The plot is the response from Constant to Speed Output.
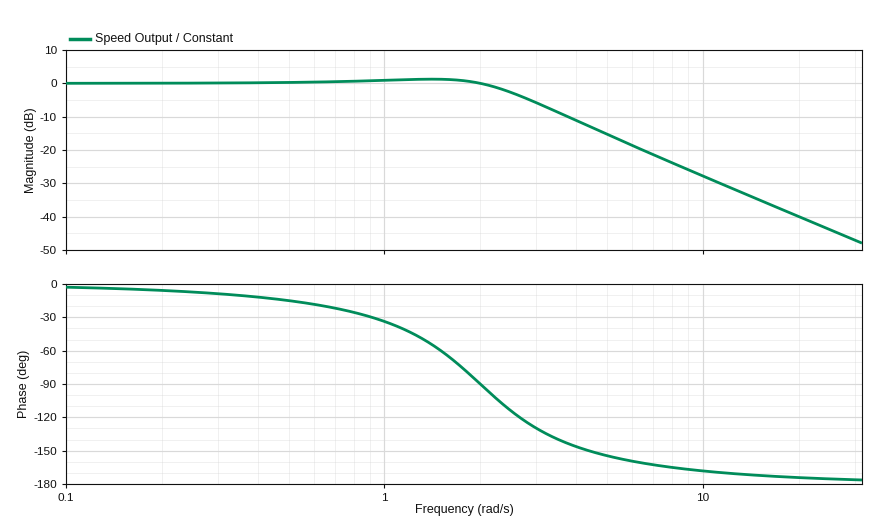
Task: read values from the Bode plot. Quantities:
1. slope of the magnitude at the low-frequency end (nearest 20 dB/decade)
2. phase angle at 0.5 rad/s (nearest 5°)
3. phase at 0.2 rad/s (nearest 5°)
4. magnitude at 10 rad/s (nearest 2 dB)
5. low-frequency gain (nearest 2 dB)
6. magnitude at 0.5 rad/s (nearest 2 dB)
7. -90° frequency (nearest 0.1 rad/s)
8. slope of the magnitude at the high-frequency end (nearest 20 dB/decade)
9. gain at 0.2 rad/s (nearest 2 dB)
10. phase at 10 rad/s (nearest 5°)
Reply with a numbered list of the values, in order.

1. 0 dB/decade
2. -15°
3. -5°
4. -28 dB
5. 0 dB
6. 0 dB
7. 2.0 rad/s
8. -40 dB/decade
9. 0 dB
10. -170°
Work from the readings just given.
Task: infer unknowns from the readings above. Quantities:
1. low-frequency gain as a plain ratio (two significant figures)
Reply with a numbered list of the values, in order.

1. 1.0
